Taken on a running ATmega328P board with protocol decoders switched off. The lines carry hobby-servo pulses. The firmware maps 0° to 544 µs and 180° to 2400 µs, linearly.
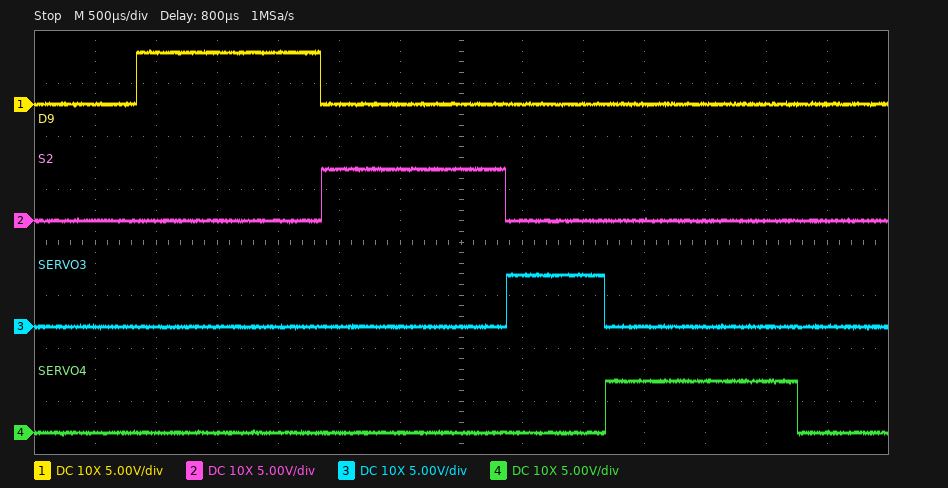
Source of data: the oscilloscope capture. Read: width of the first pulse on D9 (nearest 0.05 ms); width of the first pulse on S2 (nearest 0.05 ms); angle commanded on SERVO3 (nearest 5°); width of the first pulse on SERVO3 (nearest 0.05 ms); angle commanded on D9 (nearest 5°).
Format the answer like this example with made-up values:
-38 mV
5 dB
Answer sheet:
1.50 ms
1.50 ms
25°
0.80 ms
95°
